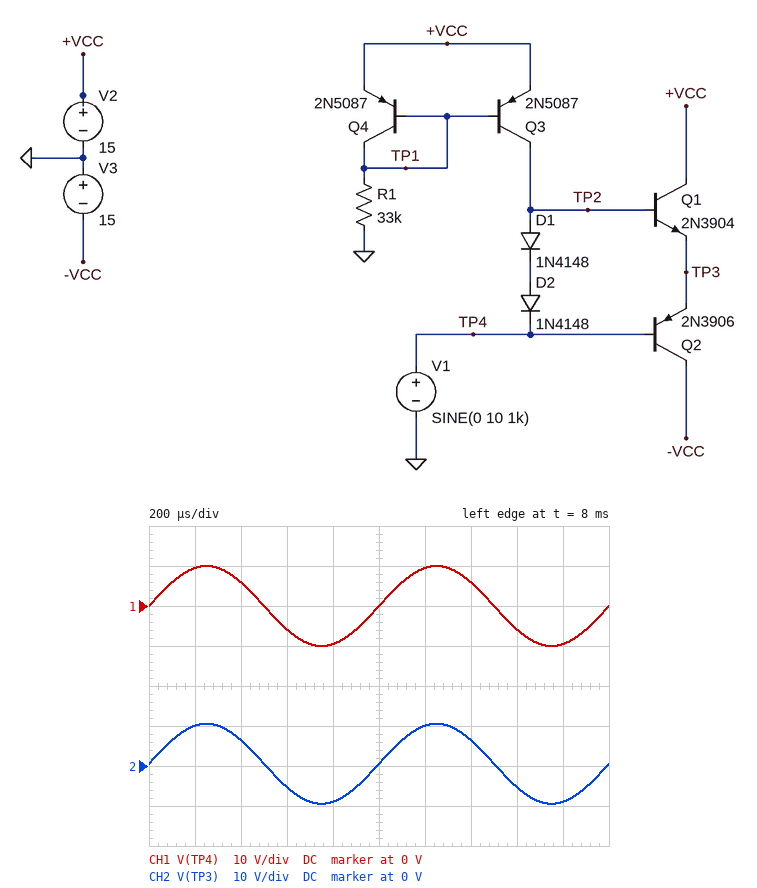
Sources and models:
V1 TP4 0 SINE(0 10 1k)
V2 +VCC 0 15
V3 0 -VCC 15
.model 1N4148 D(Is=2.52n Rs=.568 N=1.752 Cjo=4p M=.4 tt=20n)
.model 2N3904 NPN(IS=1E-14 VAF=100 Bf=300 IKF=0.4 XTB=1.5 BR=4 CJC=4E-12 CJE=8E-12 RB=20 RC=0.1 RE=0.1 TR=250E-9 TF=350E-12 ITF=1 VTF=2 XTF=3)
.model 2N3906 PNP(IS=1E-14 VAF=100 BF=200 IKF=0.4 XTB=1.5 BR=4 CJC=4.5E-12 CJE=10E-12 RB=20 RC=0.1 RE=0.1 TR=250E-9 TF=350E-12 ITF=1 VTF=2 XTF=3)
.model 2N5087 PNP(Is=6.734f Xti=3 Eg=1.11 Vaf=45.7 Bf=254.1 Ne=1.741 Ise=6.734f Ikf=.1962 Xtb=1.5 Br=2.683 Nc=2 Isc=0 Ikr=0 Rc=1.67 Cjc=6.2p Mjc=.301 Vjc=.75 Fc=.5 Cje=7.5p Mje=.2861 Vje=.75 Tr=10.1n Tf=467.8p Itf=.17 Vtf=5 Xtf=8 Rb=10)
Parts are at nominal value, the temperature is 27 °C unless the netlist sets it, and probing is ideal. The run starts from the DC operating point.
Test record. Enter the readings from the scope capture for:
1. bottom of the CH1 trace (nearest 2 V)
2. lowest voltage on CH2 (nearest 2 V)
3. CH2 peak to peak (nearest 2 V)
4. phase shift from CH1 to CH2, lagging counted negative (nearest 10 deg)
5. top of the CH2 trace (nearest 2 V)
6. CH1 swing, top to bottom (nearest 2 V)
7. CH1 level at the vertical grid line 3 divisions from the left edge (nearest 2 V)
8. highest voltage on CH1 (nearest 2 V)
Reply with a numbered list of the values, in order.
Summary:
1. -10 V
2. -10 V
3. 20 V
4. 0 deg
5. 10 V
6. 20 V
7. -6 V
8. 10 V
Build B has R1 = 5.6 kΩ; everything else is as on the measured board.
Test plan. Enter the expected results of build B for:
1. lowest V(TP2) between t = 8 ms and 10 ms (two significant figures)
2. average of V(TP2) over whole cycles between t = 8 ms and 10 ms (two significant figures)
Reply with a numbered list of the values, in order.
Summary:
1. -8.7 V
2. 1.3 V
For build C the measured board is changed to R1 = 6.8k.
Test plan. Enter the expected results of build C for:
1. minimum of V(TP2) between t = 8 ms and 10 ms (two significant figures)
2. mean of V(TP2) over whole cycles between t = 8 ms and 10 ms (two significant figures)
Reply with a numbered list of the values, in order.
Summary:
1. -8.7 V
2. 1.3 V
